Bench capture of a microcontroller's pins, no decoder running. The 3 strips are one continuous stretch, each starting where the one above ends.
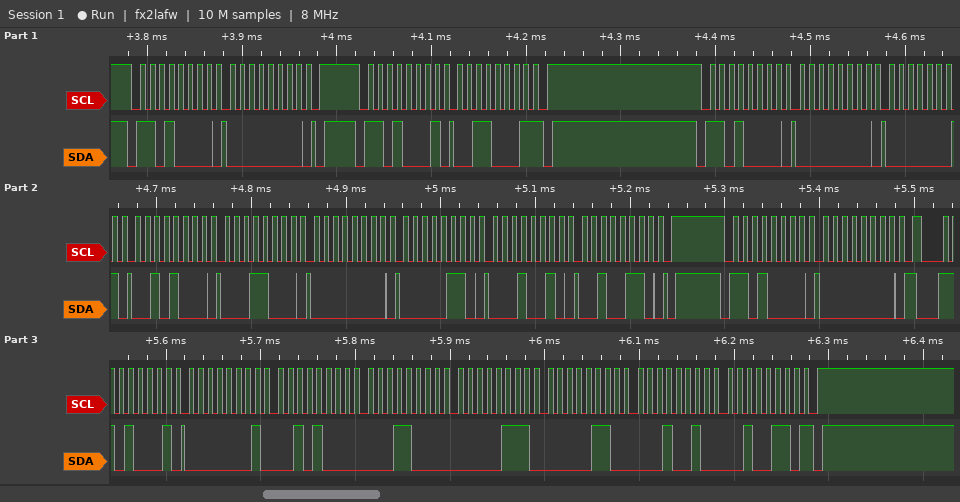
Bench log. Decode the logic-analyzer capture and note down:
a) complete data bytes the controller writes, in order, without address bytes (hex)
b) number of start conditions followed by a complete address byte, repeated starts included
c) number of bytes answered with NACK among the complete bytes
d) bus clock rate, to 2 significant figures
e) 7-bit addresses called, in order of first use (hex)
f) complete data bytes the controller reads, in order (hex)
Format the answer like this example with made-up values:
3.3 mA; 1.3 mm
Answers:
00 00 01 28 18 00 06 12 26 00; 5; 2; 100 kHz; 0x68; 31 01 28 18 07 06 12 26
